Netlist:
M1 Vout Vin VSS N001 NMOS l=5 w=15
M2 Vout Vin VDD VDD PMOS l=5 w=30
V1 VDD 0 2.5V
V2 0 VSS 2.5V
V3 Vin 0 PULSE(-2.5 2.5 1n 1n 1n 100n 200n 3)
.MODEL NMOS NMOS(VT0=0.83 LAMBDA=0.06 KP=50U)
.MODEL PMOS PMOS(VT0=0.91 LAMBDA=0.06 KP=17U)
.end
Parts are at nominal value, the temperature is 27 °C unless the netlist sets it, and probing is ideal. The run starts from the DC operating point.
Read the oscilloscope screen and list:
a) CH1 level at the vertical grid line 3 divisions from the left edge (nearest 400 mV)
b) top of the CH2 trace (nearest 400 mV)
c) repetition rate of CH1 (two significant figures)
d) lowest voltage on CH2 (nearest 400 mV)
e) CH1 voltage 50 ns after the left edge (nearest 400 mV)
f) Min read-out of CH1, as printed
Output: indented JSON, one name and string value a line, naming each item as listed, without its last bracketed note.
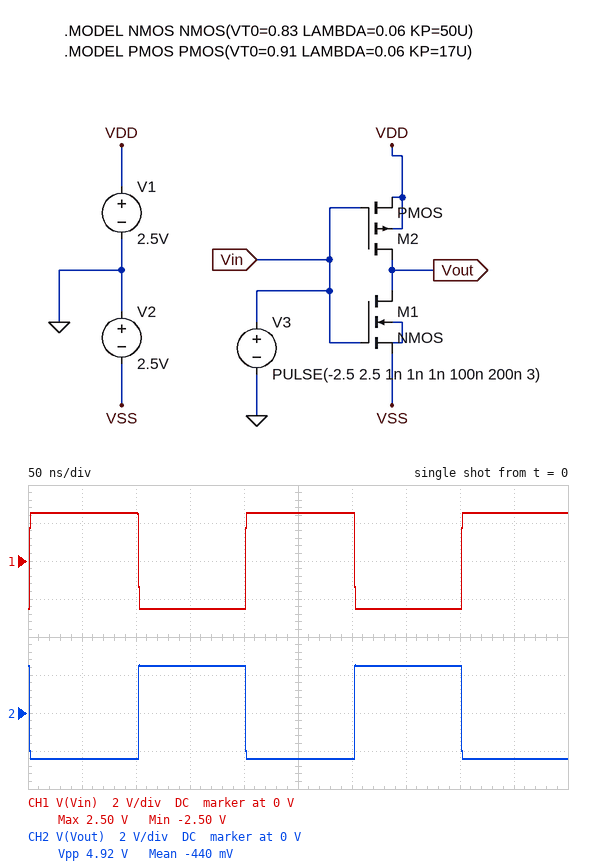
{
  "CH1 level at the vertical grid line 3 divisions from the left edge": "-2.4 V",
  "top of the CH2 trace": "2.4 V",
  "repetition rate of CH1": "5.0 MHz",
  "lowest voltage on CH2": "-2.4 V",
  "CH1 voltage 50 ns after the left edge": "2.4 V",
  "Min read-out of CH1, as printed": "-2.50 V"
}
